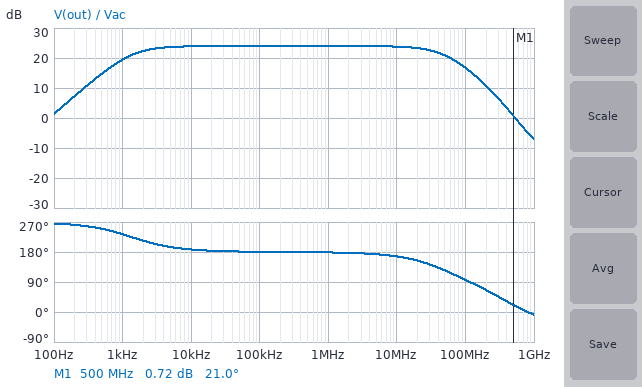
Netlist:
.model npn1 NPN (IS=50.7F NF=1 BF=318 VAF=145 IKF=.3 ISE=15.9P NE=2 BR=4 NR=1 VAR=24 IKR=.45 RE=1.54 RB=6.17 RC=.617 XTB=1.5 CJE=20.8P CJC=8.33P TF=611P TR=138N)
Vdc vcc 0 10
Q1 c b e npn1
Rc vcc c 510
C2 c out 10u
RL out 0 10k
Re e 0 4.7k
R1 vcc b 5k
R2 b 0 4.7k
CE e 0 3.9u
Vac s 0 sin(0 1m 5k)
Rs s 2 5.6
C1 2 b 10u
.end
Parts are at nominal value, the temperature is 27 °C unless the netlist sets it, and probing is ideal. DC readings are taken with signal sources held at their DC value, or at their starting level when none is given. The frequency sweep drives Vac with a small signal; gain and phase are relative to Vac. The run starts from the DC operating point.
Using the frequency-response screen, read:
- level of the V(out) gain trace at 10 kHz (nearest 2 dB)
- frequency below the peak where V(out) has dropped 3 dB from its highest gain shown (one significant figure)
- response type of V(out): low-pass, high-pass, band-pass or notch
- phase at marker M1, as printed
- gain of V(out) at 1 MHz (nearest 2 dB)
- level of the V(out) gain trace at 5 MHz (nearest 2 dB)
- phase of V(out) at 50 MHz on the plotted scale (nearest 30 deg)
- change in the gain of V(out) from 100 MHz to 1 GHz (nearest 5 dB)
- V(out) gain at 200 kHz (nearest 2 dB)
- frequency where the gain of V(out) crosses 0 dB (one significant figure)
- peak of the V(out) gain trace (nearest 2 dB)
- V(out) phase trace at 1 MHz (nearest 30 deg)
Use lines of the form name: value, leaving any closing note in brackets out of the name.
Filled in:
level of the V(out) gain trace at 10 kHz: 24 dB
frequency below the peak where V(out) has dropped 3 dB from its highest gain shown: 1 kHz
response type of V(out): low-pass, high-pass, band-pass or notch: band-pass
phase at marker M1, as printed: 21.0 deg
gain of V(out) at 1 MHz: 24 dB
level of the V(out) gain trace at 5 MHz: 24 dB
phase of V(out) at 50 MHz on the plotted scale: 120 deg
change in the gain of V(out) from 100 MHz to 1 GHz: -25 dB
V(out) gain at 200 kHz: 24 dB
frequency where the gain of V(out) crosses 0 dB: 500 MHz
peak of the V(out) gain trace: 24 dB
V(out) phase trace at 1 MHz: 180 deg
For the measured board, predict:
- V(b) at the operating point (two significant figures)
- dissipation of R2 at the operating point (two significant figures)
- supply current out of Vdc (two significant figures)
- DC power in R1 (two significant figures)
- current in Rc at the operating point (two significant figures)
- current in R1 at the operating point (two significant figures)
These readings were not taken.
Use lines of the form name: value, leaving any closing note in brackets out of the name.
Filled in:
V(b) at the operating point: 4.8 V
dissipation of R2 at the operating point: 5.0 mW
supply current out of Vdc: 1.9 mA
DC power in R1: 5.3 mW
current in Rc at the operating point: 890 µA
current in R1 at the operating point: 1.0 mA
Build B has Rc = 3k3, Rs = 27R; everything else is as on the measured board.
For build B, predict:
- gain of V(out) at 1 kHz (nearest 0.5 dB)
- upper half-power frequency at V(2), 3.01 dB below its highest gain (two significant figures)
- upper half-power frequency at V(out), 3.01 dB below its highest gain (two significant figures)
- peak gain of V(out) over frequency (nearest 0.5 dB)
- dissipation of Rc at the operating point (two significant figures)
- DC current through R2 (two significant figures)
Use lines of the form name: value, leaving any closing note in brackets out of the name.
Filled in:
gain of V(out) at 1 kHz: 33.5 dB
upper half-power frequency at V(2), 3.01 dB below its highest gain: 8.9 MHz
upper half-power frequency at V(out), 3.01 dB below its highest gain: 5.7 MHz
peak gain of V(out) over frequency: 38.0 dB
dissipation of Rc at the operating point: 2.6 mW
DC current through R2: 1.0 mA
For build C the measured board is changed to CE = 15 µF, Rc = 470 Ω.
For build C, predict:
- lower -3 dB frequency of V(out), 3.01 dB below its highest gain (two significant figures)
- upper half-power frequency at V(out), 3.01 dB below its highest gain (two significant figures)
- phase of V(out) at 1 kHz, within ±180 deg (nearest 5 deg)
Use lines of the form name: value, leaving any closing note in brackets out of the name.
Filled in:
lower -3 dB frequency of V(out), 3.01 dB below its highest gain: 350 Hz
upper half-power frequency at V(out), 3.01 dB below its highest gain: 53 MHz
phase of V(out) at 1 kHz, within ±180 deg: -160 deg
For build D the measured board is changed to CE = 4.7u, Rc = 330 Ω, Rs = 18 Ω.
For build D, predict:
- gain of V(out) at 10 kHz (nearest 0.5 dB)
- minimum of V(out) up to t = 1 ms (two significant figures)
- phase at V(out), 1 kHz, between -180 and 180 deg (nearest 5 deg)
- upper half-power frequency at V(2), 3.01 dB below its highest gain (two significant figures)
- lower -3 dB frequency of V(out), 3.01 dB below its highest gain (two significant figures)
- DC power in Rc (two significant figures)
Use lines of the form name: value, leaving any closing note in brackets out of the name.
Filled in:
gain of V(out) at 10 kHz: 20.0 dB
minimum of V(out) up to t = 1 ms: -10 mV
phase at V(out), 1 kHz, between -180 and 180 deg: -130 deg
upper half-power frequency at V(2), 3.01 dB below its highest gain: 68 MHz
lower -3 dB frequency of V(out), 3.01 dB below its highest gain: 1.1 kHz
DC power in Rc: 260 µW
